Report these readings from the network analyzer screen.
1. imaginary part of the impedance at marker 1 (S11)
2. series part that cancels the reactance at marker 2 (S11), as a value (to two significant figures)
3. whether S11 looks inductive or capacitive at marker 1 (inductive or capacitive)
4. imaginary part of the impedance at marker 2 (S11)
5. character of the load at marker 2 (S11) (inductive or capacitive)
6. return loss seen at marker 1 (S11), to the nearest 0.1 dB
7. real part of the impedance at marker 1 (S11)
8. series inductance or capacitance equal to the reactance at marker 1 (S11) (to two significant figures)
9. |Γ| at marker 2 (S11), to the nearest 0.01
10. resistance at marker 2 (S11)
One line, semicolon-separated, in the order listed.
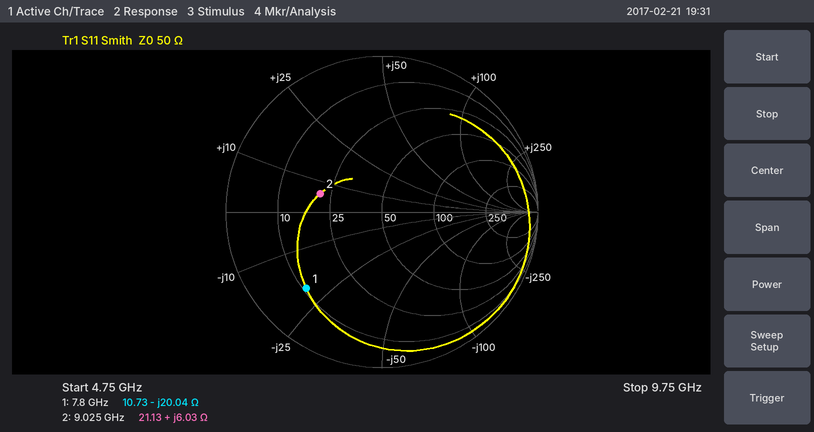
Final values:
-20.04 Ω; 2.9 pF; capacitive; +6.03 Ω; inductive; 3.2 dB; 10.73 Ω; 1.0 pF; 0.41; 21.13 Ω
